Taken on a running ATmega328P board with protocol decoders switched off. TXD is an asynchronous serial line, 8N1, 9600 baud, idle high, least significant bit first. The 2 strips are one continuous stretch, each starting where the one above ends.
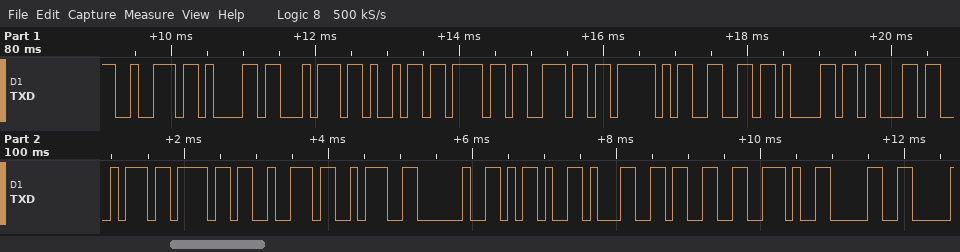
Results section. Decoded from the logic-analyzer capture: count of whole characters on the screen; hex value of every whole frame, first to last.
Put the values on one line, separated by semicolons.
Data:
20; 0x72 0x61 0x74 0x69 0x6F 0x6E 0x5F 0x66 0x61 0x63 0x74 0x6F 0x72 0x3A 0x20 0x2D 0x31 0x33 0x2E 0x30
